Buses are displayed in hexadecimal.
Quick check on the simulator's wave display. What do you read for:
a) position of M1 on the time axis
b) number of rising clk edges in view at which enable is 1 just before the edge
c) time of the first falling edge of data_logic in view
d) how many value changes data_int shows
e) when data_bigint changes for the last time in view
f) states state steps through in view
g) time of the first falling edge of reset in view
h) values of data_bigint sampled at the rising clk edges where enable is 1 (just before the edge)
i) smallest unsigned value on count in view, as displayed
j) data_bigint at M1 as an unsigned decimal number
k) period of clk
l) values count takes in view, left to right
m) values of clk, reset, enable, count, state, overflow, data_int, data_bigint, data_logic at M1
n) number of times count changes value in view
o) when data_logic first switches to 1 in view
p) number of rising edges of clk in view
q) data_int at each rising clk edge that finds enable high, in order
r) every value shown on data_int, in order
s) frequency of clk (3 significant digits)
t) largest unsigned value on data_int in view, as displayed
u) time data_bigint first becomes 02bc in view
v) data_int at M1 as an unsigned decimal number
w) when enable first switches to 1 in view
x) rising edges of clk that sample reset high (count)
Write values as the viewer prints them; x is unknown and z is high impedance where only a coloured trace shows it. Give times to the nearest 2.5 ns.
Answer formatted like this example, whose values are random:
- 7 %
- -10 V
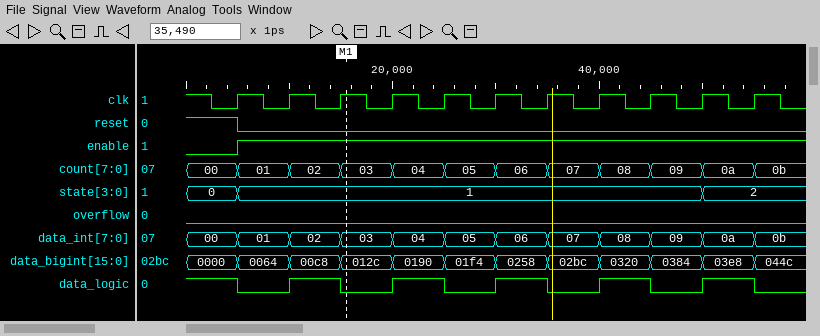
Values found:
- 15 ns
- 10
- 5 ns
- 11
- 55 ns
- 0, 1, 2
- 5 ns
- 0064, 00c8, 012c, 0190, 01f4, 0258, 02bc, 0320, 0384, 03e8
- 00
- 300
- 5 ns
- 00, 01, 02, 03, 04, 05, 06, 07, 08, 09, 0a, 0b
- clk=1, reset=0, enable=1, count=03, state=1, overflow=0, data_int=03, data_bigint=012c, data_logic=0
- 11
- 10 ns
- 11
- 01, 02, 03, 04, 05, 06, 07, 08, 09, 0a
- 00, 01, 02, 03, 04, 05, 06, 07, 08, 09, 0a, 0b
- 200 MHz
- 0b
- 35 ns
- 3
- 5 ns
- 1
